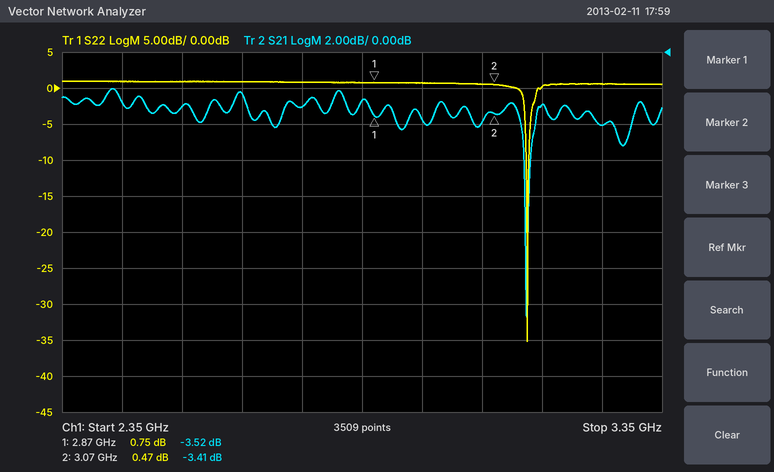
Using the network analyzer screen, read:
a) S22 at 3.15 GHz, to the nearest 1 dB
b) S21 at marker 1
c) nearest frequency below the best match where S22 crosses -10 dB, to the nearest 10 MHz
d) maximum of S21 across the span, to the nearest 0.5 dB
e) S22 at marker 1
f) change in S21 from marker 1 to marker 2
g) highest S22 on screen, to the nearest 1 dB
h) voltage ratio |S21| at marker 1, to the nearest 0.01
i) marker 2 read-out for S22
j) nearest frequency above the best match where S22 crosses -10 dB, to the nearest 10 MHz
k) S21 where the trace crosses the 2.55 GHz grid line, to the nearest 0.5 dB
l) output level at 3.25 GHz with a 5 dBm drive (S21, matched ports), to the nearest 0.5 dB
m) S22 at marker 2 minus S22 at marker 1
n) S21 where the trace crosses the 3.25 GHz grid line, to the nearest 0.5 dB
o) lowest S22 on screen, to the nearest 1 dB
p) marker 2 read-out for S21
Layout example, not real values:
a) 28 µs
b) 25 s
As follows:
a) 0 dB
b) -3.52 dB
c) 3.12 GHz
d) -2.0 dB
e) 0.75 dB
f) 0.11 dB
g) 1 dB
h) 0.67
i) 0.47 dB
j) 3.13 GHz
k) -3.0 dB
l) 1.0 dBm
m) -0.28 dB
n) -4.0 dB
o) -35 dB
p) -3.41 dB
